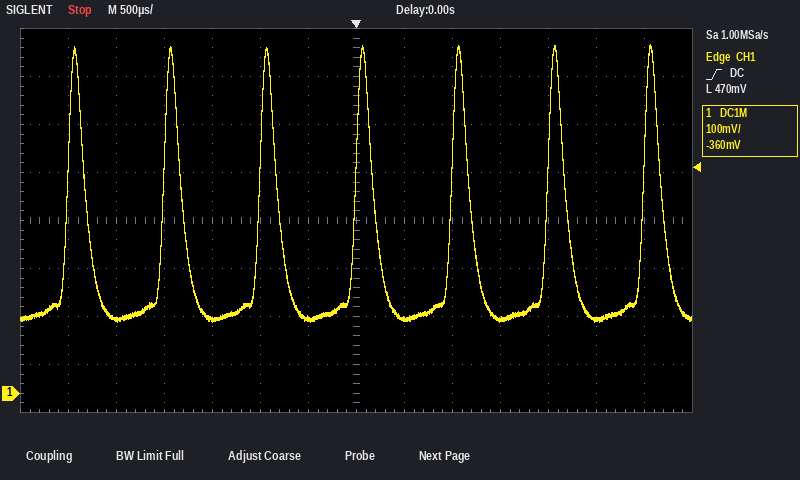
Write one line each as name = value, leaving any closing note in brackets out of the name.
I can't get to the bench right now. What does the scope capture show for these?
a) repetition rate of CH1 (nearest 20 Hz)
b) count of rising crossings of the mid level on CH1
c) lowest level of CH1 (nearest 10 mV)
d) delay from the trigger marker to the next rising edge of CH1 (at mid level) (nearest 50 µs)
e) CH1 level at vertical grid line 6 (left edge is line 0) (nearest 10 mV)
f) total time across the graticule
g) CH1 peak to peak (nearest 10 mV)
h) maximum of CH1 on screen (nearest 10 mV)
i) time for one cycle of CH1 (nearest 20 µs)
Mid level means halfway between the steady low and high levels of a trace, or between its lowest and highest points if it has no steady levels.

repetition rate of CH1 = 1.00 kHz
count of rising crossings of the mid level on CH1 = 7
lowest level of CH1 = 150 mV
delay from the trigger marker to the next rising edge of CH1 (at mid level) = 1.00 ms
CH1 level at vertical grid line 6 (left edge is line 0) = 160 mV
total time across the graticule = 7 ms
CH1 peak to peak = 580 mV
maximum of CH1 on screen = 730 mV
time for one cycle of CH1 = 1.00 ms
